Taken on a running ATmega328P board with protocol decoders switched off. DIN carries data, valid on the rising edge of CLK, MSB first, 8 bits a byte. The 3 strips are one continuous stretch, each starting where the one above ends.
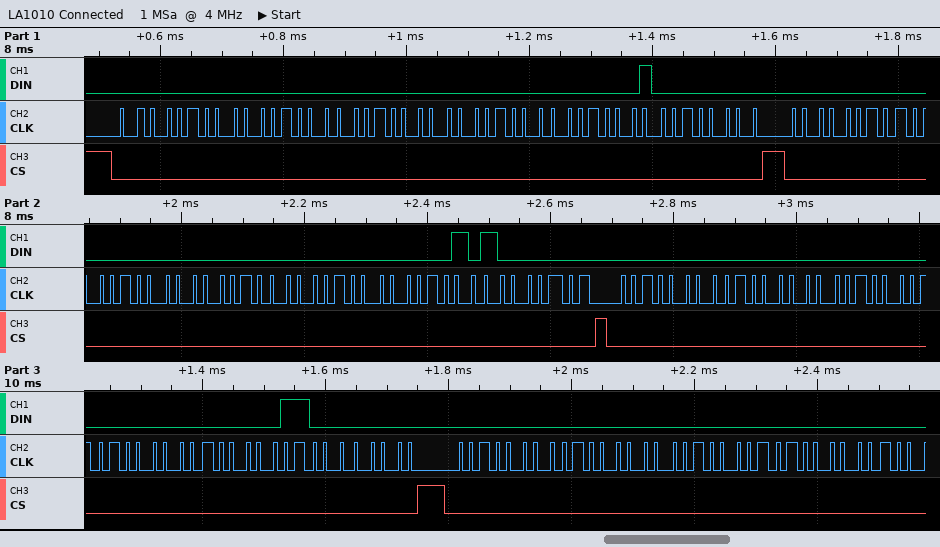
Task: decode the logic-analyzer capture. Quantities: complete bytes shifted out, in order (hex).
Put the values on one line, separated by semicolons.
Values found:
0x00 0x00 0x00 0x00 0x01 0x00 0x00 0x00 0x00 0x00 0x02 0x80 0x00 0x00 0x00 0x00 0x03 0x00 0x00 0x00 0x00 0x00
